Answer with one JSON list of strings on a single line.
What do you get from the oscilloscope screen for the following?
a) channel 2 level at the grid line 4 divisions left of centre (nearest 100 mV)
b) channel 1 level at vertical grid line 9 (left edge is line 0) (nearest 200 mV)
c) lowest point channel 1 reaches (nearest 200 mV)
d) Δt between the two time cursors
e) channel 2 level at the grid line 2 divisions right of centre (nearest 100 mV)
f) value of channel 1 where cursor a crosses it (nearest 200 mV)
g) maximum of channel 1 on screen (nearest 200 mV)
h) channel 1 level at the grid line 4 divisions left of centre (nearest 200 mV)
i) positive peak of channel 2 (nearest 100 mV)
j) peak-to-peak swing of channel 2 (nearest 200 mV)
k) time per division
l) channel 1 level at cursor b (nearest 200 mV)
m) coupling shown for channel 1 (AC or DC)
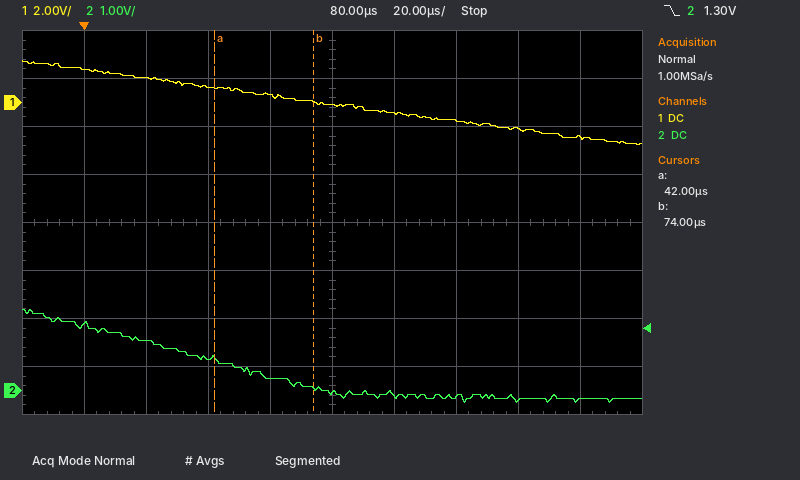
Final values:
["1.4 V", "-1.4 V", "-1.8 V", "32 µs", "-100 mV", "600 mV", "1.8 V", "1.4 V", "1.7 V", "2.0 V", "20 µs", "0.0 V", "DC"]
